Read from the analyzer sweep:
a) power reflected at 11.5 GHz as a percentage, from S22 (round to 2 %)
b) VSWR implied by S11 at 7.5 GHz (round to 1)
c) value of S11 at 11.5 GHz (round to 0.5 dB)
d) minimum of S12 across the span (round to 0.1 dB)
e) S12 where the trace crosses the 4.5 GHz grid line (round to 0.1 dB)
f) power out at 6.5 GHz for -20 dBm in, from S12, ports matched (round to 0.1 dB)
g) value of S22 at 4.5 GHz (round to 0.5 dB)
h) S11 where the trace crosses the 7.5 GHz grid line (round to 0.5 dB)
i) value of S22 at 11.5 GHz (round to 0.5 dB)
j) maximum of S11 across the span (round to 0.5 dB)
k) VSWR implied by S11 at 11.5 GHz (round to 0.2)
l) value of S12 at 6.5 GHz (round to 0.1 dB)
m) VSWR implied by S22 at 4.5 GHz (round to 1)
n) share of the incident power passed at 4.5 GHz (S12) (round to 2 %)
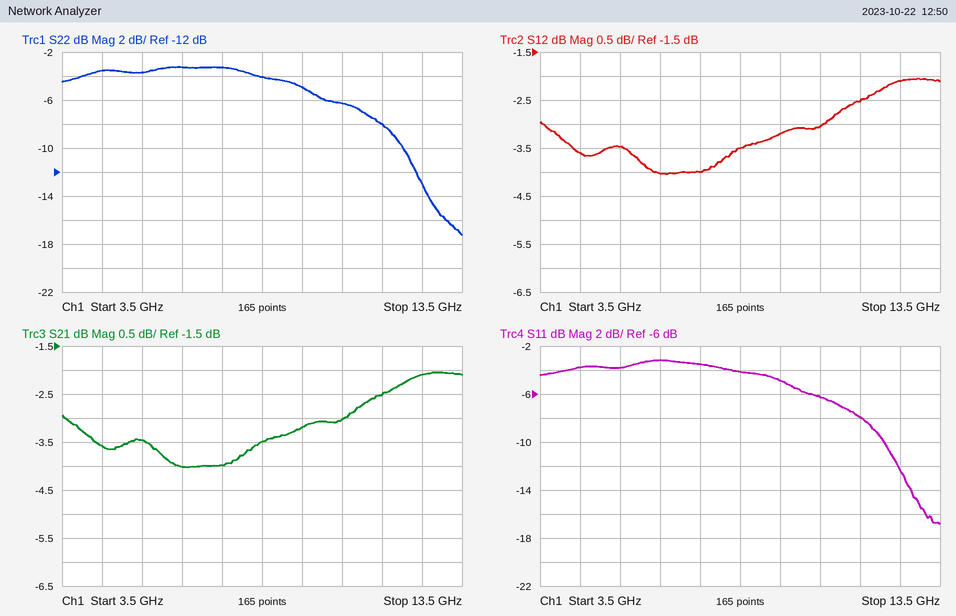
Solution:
16 %
5
-8.0 dB
-4.0 dB
-3.6 dB
-24.0 dBm
-3.5 dB
-3.5 dB
-8.0 dB
-3.0 dB
2.4
-4.0 dB
5
44 %
